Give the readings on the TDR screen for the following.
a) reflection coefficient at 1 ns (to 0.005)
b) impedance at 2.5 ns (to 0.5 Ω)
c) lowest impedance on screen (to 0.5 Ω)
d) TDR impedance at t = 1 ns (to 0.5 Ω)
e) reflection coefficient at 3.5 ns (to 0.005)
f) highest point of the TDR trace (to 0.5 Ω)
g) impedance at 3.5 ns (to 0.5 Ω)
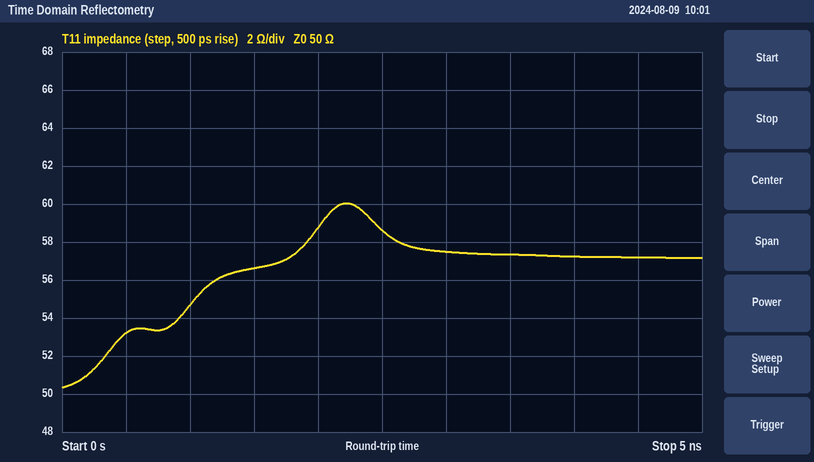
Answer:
+0.045
58.5 Ω
50.5 Ω
54.5 Ω
+0.070
60.0 Ω
57.5 Ω
